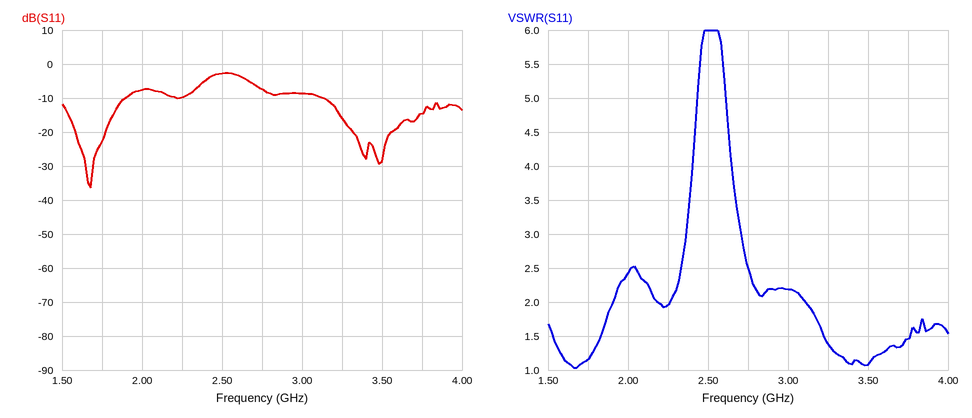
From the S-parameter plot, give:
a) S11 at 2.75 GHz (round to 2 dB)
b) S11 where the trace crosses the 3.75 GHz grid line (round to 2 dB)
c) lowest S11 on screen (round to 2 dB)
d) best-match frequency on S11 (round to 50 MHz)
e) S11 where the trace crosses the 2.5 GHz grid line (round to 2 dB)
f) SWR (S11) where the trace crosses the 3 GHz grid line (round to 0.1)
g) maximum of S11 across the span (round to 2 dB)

-8 dB
-14 dB
-36 dB
1.70 GHz
-2 dB
2.2
-2 dB
